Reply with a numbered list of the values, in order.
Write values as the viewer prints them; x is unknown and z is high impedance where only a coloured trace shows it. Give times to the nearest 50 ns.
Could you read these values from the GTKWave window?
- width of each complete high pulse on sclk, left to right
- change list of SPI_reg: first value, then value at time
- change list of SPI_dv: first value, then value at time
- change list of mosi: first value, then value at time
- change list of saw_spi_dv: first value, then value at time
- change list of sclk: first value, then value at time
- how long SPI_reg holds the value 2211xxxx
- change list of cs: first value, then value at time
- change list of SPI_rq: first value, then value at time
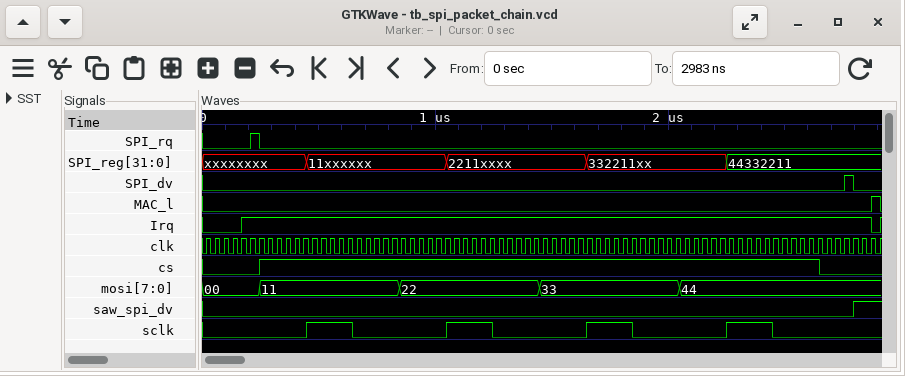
1. 200 ns, 200 ns, 200 ns, 200 ns
2. xxxxxxxx, 11xxxxxx at 450 ns, 2211xxxx at 1050 ns, 332211xx at 1650 ns, 44332211 at 2250 ns
3. 0, 1 at 2750 ns, 0 at 2800 ns
4. 00, 11 at 250 ns, 22 at 850 ns, 33 at 1450 ns, 44 at 2050 ns
5. 0, 1 at 2800 ns
6. 0, 1 at 450 ns, 0 at 650 ns, 1 at 1050 ns, 0 at 1250 ns, 1 at 1650 ns, 0 at 1850 ns, 1 at 2250 ns, 0 at 2450 ns
7. 600 ns
8. 0, 1 at 250 ns, 0 at 2650 ns
9. 0, 1 at 200 ns, 0 at 250 ns
